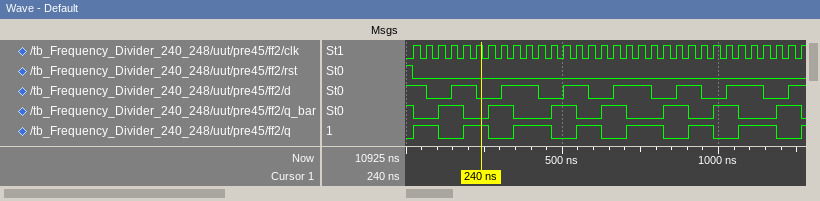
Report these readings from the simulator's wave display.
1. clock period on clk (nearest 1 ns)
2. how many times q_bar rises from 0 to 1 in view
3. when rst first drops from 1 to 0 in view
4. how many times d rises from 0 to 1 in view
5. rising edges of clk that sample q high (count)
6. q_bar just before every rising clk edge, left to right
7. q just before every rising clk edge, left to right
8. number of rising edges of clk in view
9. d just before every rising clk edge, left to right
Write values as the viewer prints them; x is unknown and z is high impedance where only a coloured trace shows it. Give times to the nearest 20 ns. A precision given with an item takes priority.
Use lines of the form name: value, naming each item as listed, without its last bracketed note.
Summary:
clock period on clk: 40 ns
how many times q_bar rises from 0 to 1 in view: 7
when rst first drops from 1 to 0 in view: 20 ns
how many times d rises from 0 to 1 in view: 7
rising edges of clk that sample q high: 17
q_bar just before every rising clk edge, left to right: 1 0 0 1 1 0 0 1 1 0 0 0 1 1 0 0 1 1 0 0 0 1 1 0 0 1 1 0 0 0 1 1
q just before every rising clk edge, left to right: 0 1 1 0 0 1 1 0 0 1 1 1 0 0 1 1 0 0 1 1 1 0 0 1 1 0 0 1 1 1 0 0
number of rising edges of clk in view: 32
d just before every rising clk edge, left to right: 1 1 0 0 1 1 0 0 1 1 1 0 0 1 1 0 0 1 1 1 0 0 1 1 0 0 1 1 1 0 0 1
